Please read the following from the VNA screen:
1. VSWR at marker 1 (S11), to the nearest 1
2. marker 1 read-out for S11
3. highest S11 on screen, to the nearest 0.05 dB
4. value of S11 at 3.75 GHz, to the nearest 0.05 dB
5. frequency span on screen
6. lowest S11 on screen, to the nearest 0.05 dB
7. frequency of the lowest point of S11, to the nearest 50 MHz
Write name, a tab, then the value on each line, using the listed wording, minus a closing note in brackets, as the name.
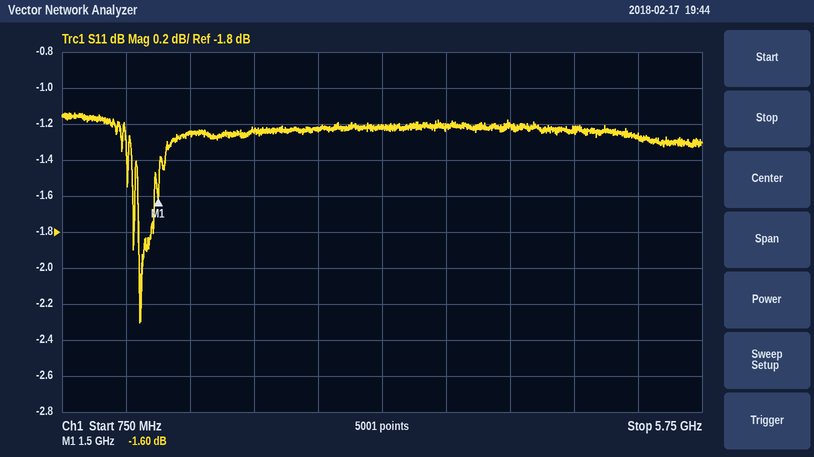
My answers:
VSWR at marker 1 (S11), to the nearest 1	11
marker 1 read-out for S11	-1.60 dB
highest S11 on screen, to the nearest 0.05 dB	-1.15 dB
value of S11 at 3.75 GHz, to the nearest 0.05 dB	-1.20 dB
frequency span on screen	5 GHz
lowest S11 on screen, to the nearest 0.05 dB	-2.30 dB
frequency of the lowest point of S11, to the nearest 50 MHz	1.35 GHz
